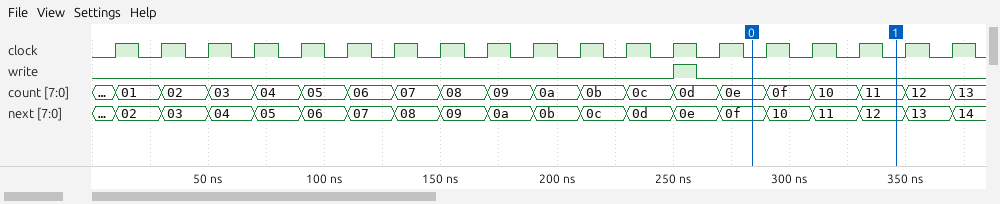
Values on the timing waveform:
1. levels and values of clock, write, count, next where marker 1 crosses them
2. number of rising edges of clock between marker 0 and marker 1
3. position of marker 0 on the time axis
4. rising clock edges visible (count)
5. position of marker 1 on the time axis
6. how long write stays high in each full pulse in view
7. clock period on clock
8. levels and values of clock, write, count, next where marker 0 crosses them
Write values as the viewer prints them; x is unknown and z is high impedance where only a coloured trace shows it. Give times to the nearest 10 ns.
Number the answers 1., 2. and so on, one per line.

1. clock=0, write=0, count=11, next=12
2. 3
3. 280 ns
4. 19
5. 350 ns
6. 10 ns
7. 20 ns
8. clock=0, write=0, count=0e, next=0f
